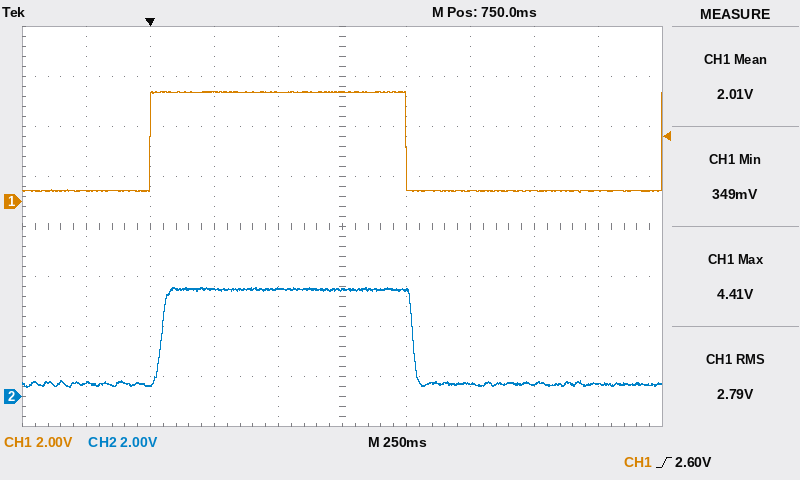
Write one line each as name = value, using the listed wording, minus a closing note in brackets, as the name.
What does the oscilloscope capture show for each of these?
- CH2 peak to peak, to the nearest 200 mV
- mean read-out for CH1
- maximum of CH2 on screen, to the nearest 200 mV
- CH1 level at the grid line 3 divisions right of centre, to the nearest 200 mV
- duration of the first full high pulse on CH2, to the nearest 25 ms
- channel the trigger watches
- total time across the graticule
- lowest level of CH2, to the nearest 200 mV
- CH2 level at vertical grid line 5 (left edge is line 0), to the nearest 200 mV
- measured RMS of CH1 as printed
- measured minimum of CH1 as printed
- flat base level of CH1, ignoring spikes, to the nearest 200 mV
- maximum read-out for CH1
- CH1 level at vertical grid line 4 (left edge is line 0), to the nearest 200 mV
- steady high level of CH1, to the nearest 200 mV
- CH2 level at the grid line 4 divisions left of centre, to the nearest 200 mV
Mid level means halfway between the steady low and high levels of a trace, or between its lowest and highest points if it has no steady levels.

CH2 peak to peak, to the nearest 200 mV = 4.0 V
mean read-out for CH1 = 2.01 V
maximum of CH2 on screen, to the nearest 200 mV = 4.4 V
CH1 level at the grid line 3 divisions right of centre, to the nearest 200 mV = 400 mV
duration of the first full high pulse on CH2, to the nearest 25 ms = 975 ms
channel the trigger watches = CH1
total time across the graticule = 2.5 s
lowest level of CH2, to the nearest 200 mV = 400 mV
CH2 level at vertical grid line 5 (left edge is line 0), to the nearest 200 mV = 4.2 V
measured RMS of CH1 as printed = 2.79 V
measured minimum of CH1 as printed = 349 mV
flat base level of CH1, ignoring spikes, to the nearest 200 mV = 400 mV
maximum read-out for CH1 = 4.41 V
CH1 level at vertical grid line 4 (left edge is line 0), to the nearest 200 mV = 4.4 V
steady high level of CH1, to the nearest 200 mV = 4.4 V
CH2 level at the grid line 4 divisions left of centre, to the nearest 200 mV = 600 mV
